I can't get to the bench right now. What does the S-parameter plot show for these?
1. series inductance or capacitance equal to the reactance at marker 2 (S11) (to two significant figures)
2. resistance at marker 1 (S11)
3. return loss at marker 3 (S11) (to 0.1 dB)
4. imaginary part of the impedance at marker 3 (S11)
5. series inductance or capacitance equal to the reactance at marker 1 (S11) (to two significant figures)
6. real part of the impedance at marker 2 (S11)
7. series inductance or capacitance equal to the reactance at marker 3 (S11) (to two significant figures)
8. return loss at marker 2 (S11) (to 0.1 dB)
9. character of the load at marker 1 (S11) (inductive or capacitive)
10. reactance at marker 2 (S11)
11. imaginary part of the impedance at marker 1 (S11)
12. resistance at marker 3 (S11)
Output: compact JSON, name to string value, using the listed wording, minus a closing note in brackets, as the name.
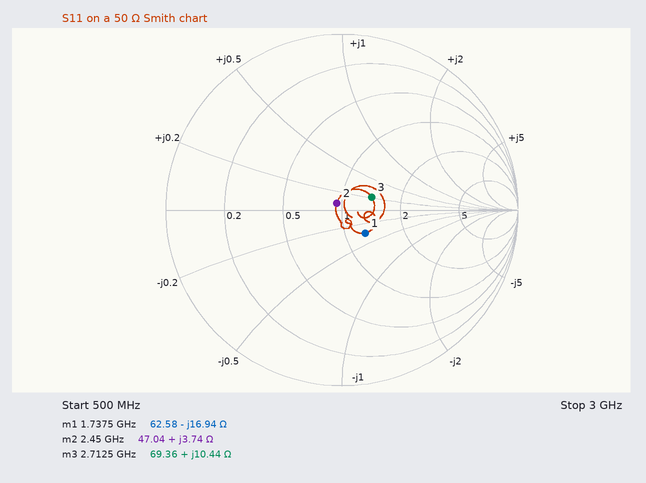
{"series inductance or capacitance equal to the reactance at marker 2 (S11)": "240 pH", "resistance at marker 1": "62.58 Ω", "return loss at marker 3 (S11)": "14.7 dB", "imaginary part of the impedance at marker 3": "+10.44 Ω", "series inductance or capacitance equal to the reactance at marker 1 (S11)": "5.4 pF", "real part of the impedance at marker 2": "47.04 Ω", "series inductance or capacitance equal to the reactance at marker 3 (S11)": "610 pH", "return loss at marker 2 (S11)": "26.2 dB", "character of the load at marker 1 (S11)": "capacitive", "reactance at marker 2": "+3.74 Ω", "imaginary part of the impedance at marker 1": "-16.94 Ω", "resistance at marker 3": "69.36 Ω"}
